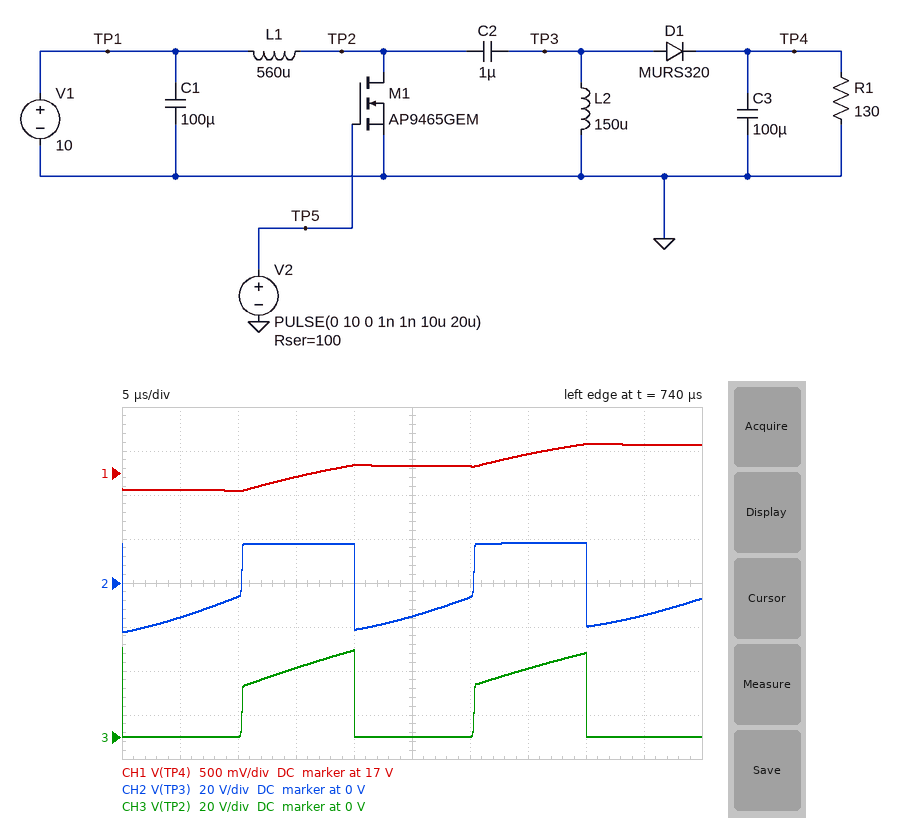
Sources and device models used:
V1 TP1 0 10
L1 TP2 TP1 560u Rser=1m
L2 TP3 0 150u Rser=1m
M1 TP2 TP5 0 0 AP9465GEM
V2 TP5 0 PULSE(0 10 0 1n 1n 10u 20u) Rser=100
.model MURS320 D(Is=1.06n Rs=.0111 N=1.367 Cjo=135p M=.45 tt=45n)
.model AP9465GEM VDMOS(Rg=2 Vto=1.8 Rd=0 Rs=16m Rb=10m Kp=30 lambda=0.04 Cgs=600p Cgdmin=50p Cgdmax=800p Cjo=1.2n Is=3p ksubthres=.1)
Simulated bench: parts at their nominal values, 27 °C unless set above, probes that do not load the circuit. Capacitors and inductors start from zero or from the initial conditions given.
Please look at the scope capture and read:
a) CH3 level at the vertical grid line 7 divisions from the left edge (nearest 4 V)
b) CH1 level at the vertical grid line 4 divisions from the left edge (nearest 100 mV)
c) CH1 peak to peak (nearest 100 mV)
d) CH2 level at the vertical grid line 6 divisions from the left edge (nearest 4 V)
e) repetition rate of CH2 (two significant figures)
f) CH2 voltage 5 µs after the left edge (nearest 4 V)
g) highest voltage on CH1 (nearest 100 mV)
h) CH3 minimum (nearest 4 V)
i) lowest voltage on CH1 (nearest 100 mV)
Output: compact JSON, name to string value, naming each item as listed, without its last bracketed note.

{"CH3 level at the vertical grid line 7 divisions from the left edge": "32 V", "CH1 level at the vertical grid line 4 divisions from the left edge": "17.1 V", "CH1 peak to peak": "500 mV", "CH2 level at the vertical grid line 6 divisions from the left edge": "-8 V", "repetition rate of CH2": "50 kHz", "CH2 voltage 5 µs after the left edge": "-16 V", "highest voltage on CH1": "17.3 V", "CH3 minimum": "0 V", "lowest voltage on CH1": "16.8 V"}
